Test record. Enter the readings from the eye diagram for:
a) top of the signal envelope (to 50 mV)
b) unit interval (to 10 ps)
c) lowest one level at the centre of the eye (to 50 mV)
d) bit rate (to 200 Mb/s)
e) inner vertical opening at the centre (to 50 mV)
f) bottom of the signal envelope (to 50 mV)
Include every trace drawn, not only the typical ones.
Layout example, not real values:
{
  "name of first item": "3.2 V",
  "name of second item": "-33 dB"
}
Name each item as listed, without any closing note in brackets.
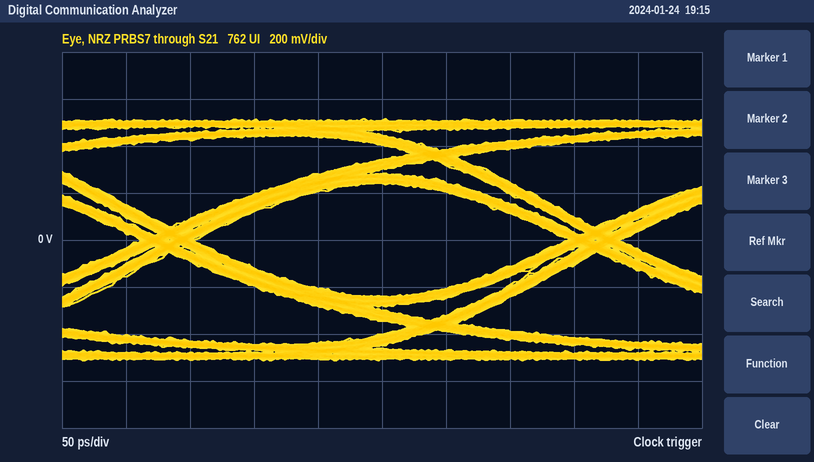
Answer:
{
  "top of the signal envelope": "500 mV",
  "unit interval": "330 ps",
  "lowest one level at the centre of the eye": "250 mV",
  "bit rate": "3.0 Gb/s",
  "inner vertical opening at the centre": "500 mV",
  "bottom of the signal envelope": "-500 mV"
}
